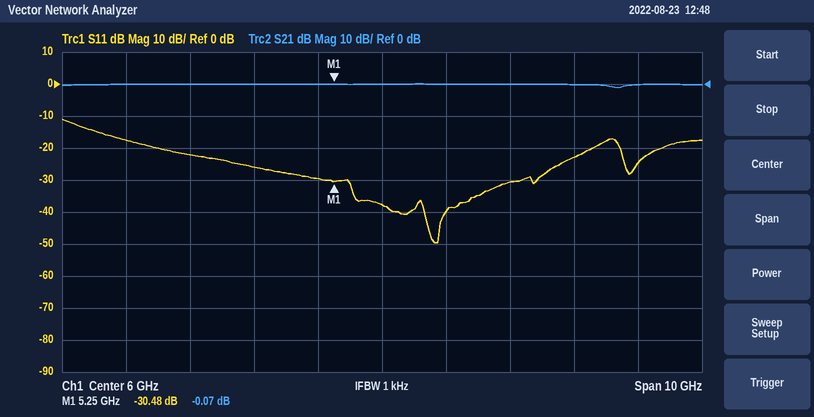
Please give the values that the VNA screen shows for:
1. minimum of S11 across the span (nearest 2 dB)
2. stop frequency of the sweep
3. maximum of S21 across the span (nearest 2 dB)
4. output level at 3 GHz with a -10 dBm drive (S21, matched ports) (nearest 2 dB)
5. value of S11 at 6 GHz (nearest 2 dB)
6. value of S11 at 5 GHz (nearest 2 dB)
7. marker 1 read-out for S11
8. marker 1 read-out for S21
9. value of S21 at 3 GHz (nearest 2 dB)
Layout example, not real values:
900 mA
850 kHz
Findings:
-50 dB
11 GHz
0 dB
-10 dBm
-38 dB
-30 dB
-30.48 dB
-0.07 dB
0 dB
